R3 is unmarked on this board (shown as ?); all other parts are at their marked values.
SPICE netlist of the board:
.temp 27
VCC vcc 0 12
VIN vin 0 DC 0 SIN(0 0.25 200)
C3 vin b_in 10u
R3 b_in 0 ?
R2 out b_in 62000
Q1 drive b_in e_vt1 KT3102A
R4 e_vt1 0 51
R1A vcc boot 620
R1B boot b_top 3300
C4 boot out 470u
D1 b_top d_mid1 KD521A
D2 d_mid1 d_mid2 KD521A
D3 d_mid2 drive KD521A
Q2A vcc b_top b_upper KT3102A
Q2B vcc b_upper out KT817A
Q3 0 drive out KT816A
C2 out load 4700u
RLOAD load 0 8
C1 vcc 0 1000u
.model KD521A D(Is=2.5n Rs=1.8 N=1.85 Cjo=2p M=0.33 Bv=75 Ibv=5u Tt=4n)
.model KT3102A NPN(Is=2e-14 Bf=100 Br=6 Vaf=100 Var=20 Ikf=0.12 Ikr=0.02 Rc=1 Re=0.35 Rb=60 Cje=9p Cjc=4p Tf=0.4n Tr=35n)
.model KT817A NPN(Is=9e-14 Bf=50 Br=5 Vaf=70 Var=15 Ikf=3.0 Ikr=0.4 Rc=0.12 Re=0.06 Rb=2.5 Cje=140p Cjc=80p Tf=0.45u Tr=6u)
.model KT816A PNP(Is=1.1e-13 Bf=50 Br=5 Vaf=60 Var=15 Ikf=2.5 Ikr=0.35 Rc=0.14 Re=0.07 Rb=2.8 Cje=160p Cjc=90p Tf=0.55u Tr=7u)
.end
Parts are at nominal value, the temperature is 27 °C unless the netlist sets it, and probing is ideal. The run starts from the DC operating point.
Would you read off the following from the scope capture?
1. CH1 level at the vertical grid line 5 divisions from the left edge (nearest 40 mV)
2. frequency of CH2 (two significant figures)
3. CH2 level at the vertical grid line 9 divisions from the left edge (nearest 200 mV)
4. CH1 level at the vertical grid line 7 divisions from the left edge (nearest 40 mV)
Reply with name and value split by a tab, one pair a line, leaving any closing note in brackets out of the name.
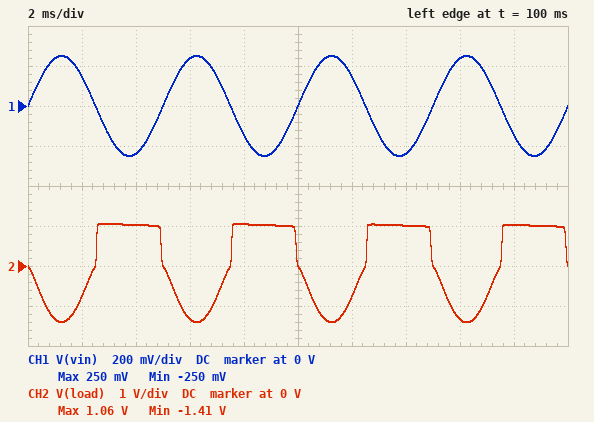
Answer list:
CH1 level at the vertical grid line 5 divisions from the left edge	0 V
frequency of CH2	200 Hz
CH2 level at the vertical grid line 9 divisions from the left edge	1.0 V
CH1 level at the vertical grid line 7 divisions from the left edge	-240 mV
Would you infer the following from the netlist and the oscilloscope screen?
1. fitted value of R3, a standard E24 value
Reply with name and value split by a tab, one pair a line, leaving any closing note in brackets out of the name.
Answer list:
fitted value of R3, a standard E24 value	4.3 kΩ
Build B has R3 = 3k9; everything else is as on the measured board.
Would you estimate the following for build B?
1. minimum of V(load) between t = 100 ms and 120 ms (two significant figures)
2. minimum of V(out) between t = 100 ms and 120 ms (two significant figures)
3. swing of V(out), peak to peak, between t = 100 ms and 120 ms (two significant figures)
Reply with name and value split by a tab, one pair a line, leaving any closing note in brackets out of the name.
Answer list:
minimum of V(load) between t = 100 ms and 120 ms	-1.2 V
minimum of V(out) between t = 100 ms and 120 ms	9.2 V
swing of V(out), peak to peak, between t = 100 ms and 120 ms	2.0 V
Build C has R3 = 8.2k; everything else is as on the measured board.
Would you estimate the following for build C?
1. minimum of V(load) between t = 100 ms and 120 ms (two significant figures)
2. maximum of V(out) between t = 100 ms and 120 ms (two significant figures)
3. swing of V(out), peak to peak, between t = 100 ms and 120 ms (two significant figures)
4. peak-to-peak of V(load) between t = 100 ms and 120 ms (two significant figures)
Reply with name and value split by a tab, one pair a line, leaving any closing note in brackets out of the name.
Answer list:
minimum of V(load) between t = 100 ms and 120 ms	-2.2 V
maximum of V(out) between t = 100 ms and 120 ms	11 V
swing of V(out), peak to peak, between t = 100 ms and 120 ms	4.9 V
peak-to-peak of V(load) between t = 100 ms and 120 ms	5.0 V
